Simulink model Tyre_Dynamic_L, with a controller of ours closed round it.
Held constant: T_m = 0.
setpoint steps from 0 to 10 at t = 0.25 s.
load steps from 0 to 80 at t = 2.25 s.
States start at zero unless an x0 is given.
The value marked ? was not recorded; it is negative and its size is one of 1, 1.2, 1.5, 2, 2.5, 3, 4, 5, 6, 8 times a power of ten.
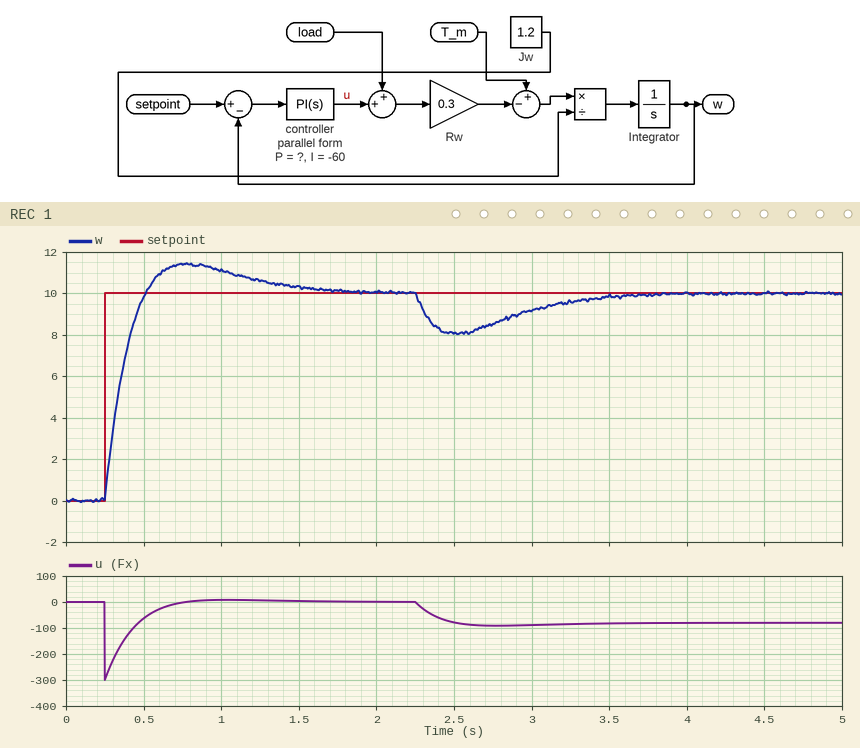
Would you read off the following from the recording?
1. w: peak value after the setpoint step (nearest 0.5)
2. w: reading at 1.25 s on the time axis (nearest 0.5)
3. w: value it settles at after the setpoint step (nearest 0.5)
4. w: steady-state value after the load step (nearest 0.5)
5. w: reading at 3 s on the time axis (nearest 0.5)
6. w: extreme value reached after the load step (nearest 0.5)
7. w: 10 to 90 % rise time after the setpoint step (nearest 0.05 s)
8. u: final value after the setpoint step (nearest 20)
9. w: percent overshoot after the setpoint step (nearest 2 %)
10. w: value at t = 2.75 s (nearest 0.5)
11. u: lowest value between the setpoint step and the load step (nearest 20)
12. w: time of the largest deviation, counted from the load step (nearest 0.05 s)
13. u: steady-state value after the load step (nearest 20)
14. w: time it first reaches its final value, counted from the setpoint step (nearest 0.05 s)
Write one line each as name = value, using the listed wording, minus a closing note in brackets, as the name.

w: peak value after the setpoint step = 11.5
w: reading at 1.25 s on the time axis = 10.5
w: value it settles at after the setpoint step = 10.0
w: steady-state value after the load step = 10.0
w: reading at 3 s on the time axis = 9.0
w: extreme value reached after the load step = 8.0
w: 10 to 90 % rise time after the setpoint step = 0.20 s
u: final value after the setpoint step = 0
w: percent overshoot after the setpoint step = 14 %
w: value at t = 2.75 s = 8.5
u: lowest value between the setpoint step and the load step = -300
w: time of the largest deviation, counted from the load step = 0.25 s
u: steady-state value after the load step = -80
w: time it first reaches its final value, counted from the setpoint step = 0.25 s
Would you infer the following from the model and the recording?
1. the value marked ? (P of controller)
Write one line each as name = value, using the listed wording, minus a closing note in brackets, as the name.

the value marked ? = -30
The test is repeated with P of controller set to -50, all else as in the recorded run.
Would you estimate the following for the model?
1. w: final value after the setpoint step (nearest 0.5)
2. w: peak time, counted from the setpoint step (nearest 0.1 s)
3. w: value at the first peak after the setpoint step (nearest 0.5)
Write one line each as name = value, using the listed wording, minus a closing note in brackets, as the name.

w: final value after the setpoint step = 10.0
w: peak time, counted from the setpoint step = 0.4 s
w: value at the first peak after the setpoint step = 10.5
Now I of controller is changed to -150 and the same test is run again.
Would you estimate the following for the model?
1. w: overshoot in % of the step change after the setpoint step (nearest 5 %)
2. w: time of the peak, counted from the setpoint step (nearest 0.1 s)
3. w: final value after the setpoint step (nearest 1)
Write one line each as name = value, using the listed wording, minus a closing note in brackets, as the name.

w: overshoot in % of the step change after the setpoint step = 25 %
w: time of the peak, counted from the setpoint step = 0.4 s
w: final value after the setpoint step = 10
